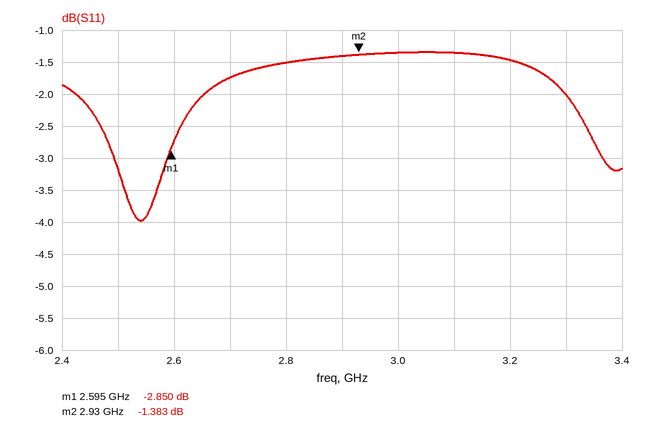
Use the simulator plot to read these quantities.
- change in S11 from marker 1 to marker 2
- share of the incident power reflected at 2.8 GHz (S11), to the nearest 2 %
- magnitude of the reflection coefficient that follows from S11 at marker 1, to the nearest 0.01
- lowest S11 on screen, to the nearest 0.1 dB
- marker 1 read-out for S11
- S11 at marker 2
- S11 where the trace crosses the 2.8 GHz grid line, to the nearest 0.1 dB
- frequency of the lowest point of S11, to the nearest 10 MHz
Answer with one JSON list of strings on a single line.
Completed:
["1.467 dB", "70 %", "0.72", "-4.0 dB", "-2.850 dB", "-1.383 dB", "-1.5 dB", "2.54 GHz"]
